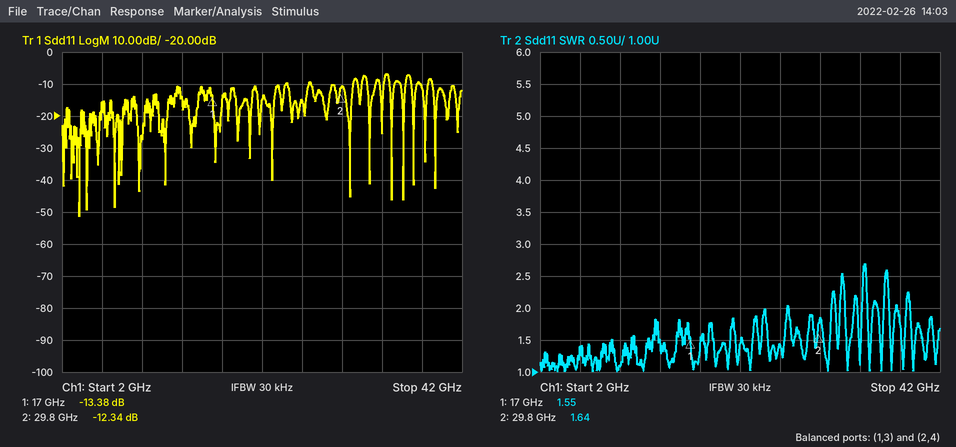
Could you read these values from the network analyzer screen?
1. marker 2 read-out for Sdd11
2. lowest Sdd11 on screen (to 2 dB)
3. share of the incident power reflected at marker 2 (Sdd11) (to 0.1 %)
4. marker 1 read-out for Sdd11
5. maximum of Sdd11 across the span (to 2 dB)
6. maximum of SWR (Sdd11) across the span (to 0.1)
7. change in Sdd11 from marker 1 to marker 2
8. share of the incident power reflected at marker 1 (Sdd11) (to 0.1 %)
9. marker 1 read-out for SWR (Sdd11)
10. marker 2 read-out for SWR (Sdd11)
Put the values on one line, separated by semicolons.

-12.34 dB; -52 dB; 5.8 %; -13.38 dB; -6 dB; 2.7; 1.04 dB; 4.6 %; 1.55; 1.64
